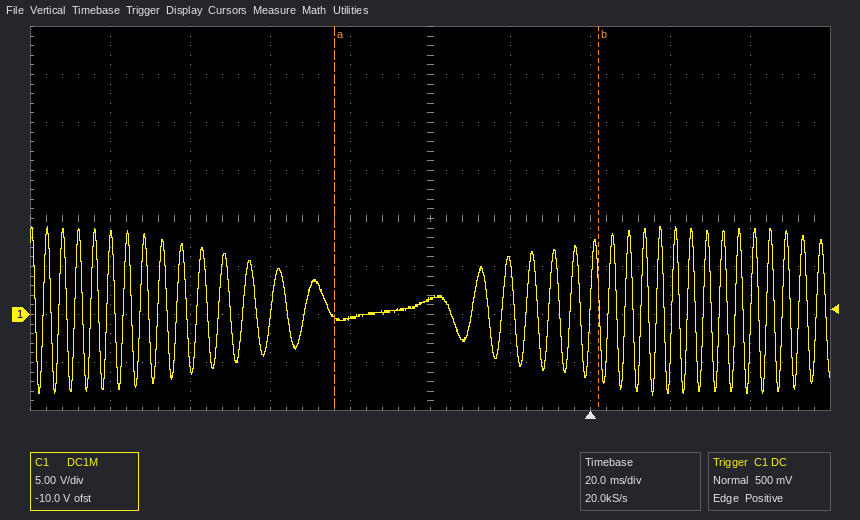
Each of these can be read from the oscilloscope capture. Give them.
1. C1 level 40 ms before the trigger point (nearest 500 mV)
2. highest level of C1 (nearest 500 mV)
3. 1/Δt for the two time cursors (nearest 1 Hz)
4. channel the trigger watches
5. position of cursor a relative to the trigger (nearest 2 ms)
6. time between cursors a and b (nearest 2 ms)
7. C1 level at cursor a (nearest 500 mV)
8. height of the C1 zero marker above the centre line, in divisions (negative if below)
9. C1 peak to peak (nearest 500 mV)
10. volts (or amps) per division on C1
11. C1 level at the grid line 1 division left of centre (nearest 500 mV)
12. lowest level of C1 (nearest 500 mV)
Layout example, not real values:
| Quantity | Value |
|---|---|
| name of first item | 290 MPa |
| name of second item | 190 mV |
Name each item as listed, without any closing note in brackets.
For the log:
| Quantity | Value |
|---|---|
| C1 level 40 ms before the trigger point | 1.5 V |
| highest level of C1 | 9.0 V |
| 1/Δt for the two time cursors | 15 Hz |
| channel the trigger watches | C1 |
| position of cursor a relative to the trigger | -64 ms |
| time between cursors a and b | 66 ms |
| C1 level at cursor a | -500 mV |
| height of the C1 zero marker above the centre line, in divisions | -2.0 div |
| C1 peak to peak | 17.5 V |
| volts (or amps) per division on C1 | 5 V |
| C1 level at the grid line 1 division left of centre | -500 mV |
| lowest level of C1 | -8.5 V |
